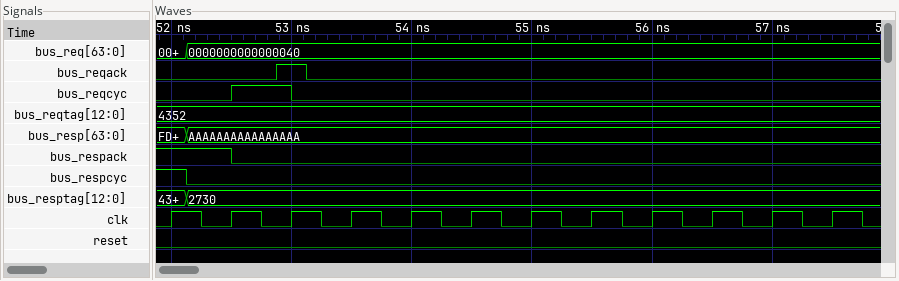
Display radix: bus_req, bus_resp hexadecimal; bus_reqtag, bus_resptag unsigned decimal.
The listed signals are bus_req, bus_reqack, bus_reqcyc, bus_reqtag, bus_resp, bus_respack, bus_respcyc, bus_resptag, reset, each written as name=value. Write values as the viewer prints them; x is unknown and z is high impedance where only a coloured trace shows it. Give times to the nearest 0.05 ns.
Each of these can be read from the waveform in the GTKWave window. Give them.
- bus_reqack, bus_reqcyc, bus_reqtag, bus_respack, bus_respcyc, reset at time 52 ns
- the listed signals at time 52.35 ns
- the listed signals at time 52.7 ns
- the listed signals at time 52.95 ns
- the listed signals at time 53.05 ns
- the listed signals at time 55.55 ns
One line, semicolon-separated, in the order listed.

bus_reqack=0, bus_reqcyc=0, bus_reqtag=4352, bus_respack=1, bus_respcyc=1, reset=0; bus_req=0000000000000040, bus_reqack=0, bus_reqcyc=0, bus_reqtag=4352, bus_resp=AAAAAAAAAAAAAAAA, bus_respack=1, bus_respcyc=0, bus_resptag=2730, reset=0; bus_req=0000000000000040, bus_reqack=0, bus_reqcyc=1, bus_reqtag=4352, bus_resp=AAAAAAAAAAAAAAAA, bus_respack=0, bus_respcyc=0, bus_resptag=2730, reset=0; bus_req=0000000000000040, bus_reqack=1, bus_reqcyc=1, bus_reqtag=4352, bus_resp=AAAAAAAAAAAAAAAA, bus_respack=0, bus_respcyc=0, bus_resptag=2730, reset=0; bus_req=0000000000000040, bus_reqack=1, bus_reqcyc=0, bus_reqtag=4352, bus_resp=AAAAAAAAAAAAAAAA, bus_respack=0, bus_respcyc=0, bus_resptag=2730, reset=0; bus_req=0000000000000040, bus_reqack=0, bus_reqcyc=0, bus_reqtag=4352, bus_resp=AAAAAAAAAAAAAAAA, bus_respack=0, bus_respcyc=0, bus_resptag=2730, reset=0
